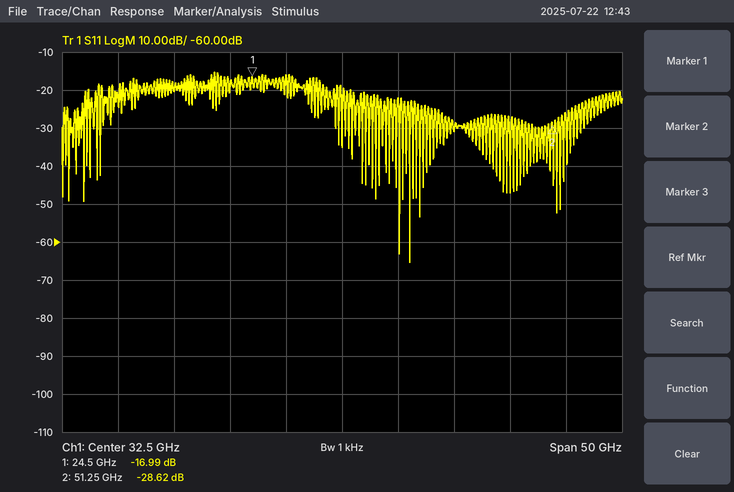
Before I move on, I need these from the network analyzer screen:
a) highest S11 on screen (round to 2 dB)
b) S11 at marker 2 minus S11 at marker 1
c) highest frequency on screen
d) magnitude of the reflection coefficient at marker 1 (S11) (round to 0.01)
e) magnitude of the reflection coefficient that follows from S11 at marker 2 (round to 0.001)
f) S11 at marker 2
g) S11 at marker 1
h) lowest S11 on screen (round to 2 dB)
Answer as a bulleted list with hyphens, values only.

- -16 dB
- -11.63 dB
- 57.5 GHz
- 0.14
- 0.037
- -28.62 dB
- -16.99 dB
- -66 dB
